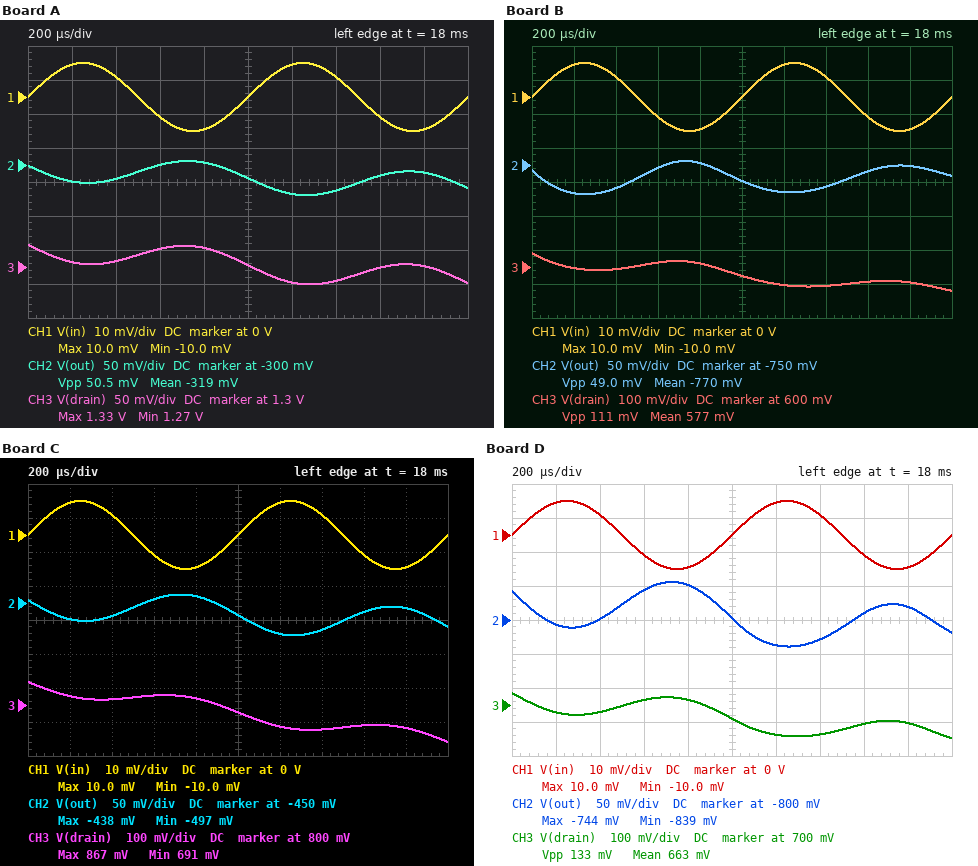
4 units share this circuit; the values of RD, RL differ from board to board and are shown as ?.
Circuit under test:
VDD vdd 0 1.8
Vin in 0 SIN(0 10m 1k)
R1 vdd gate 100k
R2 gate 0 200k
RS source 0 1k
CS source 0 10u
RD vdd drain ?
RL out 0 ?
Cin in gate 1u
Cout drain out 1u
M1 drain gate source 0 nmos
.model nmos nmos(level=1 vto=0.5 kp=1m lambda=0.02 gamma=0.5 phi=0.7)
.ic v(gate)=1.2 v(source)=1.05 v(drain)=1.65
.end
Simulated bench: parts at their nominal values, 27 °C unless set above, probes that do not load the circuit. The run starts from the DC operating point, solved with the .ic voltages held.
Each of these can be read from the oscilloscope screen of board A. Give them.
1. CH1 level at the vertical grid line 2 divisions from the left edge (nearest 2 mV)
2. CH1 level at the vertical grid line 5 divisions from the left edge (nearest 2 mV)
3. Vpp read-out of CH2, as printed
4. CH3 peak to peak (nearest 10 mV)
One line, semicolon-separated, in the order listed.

6 mV; 0 V; 50.5 mV; 60 mV
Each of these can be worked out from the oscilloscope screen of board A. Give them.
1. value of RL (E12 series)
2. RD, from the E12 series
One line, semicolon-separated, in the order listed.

27 kΩ; 5.6 kΩ
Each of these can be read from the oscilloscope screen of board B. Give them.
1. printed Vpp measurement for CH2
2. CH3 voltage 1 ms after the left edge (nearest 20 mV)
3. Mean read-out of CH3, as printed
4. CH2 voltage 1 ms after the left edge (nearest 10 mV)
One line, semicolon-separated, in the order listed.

49.0 mV; 580 mV; 577 mV; -770 mV
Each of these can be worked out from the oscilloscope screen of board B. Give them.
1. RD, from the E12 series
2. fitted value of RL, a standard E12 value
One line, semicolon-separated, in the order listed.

27 kΩ; 15 kΩ
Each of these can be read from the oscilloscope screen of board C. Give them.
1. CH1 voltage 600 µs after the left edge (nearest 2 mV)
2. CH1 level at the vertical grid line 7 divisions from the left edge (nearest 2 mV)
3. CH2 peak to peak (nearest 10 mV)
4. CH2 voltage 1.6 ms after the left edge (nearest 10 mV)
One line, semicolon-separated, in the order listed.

-6 mV; 6 mV; 60 mV; -460 mV
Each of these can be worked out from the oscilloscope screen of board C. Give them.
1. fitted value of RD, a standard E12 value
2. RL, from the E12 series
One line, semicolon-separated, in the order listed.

33 kΩ; 6.8 kΩ
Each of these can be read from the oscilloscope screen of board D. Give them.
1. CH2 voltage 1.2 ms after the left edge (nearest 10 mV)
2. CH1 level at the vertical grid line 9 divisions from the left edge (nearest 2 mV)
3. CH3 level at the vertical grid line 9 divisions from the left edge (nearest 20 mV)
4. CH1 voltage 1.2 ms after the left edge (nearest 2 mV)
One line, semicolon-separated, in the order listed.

-840 mV; -10 mV; 640 mV; 10 mV
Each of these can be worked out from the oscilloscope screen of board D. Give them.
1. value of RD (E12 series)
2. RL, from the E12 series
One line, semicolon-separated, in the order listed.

18 kΩ; 22 kΩ
